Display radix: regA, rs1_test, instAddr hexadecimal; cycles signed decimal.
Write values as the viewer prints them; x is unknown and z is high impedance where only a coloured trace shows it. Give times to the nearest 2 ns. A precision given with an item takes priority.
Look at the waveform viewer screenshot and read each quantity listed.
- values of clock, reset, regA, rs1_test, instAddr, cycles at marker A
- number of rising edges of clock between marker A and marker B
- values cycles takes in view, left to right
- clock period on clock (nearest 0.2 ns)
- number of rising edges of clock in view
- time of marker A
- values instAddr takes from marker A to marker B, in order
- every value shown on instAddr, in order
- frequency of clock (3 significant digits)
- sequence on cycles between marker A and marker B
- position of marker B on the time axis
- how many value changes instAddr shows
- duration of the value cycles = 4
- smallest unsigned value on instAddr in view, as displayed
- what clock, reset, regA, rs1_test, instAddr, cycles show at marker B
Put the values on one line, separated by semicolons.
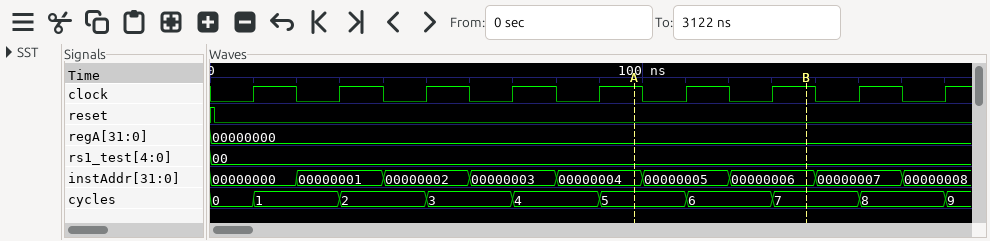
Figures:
clock=1, reset=0, regA=00000000, rs1_test=00, instAddr=00000004, cycles=5; 2; 0, 1, 2, 3, 4, 5, 6, 7, 8, 9; 20 ns; 9; 98 ns; 00000004, 00000005, 00000006; 00000000, 00000001, 00000002, 00000003, 00000004, 00000005, 00000006, 00000007, 00000008; 50.0 MHz; 5, 6, 7; 138 ns; 8; 20 ns; 00000000; clock=1, reset=0, regA=00000000, rs1_test=00, instAddr=00000006, cycles=7
